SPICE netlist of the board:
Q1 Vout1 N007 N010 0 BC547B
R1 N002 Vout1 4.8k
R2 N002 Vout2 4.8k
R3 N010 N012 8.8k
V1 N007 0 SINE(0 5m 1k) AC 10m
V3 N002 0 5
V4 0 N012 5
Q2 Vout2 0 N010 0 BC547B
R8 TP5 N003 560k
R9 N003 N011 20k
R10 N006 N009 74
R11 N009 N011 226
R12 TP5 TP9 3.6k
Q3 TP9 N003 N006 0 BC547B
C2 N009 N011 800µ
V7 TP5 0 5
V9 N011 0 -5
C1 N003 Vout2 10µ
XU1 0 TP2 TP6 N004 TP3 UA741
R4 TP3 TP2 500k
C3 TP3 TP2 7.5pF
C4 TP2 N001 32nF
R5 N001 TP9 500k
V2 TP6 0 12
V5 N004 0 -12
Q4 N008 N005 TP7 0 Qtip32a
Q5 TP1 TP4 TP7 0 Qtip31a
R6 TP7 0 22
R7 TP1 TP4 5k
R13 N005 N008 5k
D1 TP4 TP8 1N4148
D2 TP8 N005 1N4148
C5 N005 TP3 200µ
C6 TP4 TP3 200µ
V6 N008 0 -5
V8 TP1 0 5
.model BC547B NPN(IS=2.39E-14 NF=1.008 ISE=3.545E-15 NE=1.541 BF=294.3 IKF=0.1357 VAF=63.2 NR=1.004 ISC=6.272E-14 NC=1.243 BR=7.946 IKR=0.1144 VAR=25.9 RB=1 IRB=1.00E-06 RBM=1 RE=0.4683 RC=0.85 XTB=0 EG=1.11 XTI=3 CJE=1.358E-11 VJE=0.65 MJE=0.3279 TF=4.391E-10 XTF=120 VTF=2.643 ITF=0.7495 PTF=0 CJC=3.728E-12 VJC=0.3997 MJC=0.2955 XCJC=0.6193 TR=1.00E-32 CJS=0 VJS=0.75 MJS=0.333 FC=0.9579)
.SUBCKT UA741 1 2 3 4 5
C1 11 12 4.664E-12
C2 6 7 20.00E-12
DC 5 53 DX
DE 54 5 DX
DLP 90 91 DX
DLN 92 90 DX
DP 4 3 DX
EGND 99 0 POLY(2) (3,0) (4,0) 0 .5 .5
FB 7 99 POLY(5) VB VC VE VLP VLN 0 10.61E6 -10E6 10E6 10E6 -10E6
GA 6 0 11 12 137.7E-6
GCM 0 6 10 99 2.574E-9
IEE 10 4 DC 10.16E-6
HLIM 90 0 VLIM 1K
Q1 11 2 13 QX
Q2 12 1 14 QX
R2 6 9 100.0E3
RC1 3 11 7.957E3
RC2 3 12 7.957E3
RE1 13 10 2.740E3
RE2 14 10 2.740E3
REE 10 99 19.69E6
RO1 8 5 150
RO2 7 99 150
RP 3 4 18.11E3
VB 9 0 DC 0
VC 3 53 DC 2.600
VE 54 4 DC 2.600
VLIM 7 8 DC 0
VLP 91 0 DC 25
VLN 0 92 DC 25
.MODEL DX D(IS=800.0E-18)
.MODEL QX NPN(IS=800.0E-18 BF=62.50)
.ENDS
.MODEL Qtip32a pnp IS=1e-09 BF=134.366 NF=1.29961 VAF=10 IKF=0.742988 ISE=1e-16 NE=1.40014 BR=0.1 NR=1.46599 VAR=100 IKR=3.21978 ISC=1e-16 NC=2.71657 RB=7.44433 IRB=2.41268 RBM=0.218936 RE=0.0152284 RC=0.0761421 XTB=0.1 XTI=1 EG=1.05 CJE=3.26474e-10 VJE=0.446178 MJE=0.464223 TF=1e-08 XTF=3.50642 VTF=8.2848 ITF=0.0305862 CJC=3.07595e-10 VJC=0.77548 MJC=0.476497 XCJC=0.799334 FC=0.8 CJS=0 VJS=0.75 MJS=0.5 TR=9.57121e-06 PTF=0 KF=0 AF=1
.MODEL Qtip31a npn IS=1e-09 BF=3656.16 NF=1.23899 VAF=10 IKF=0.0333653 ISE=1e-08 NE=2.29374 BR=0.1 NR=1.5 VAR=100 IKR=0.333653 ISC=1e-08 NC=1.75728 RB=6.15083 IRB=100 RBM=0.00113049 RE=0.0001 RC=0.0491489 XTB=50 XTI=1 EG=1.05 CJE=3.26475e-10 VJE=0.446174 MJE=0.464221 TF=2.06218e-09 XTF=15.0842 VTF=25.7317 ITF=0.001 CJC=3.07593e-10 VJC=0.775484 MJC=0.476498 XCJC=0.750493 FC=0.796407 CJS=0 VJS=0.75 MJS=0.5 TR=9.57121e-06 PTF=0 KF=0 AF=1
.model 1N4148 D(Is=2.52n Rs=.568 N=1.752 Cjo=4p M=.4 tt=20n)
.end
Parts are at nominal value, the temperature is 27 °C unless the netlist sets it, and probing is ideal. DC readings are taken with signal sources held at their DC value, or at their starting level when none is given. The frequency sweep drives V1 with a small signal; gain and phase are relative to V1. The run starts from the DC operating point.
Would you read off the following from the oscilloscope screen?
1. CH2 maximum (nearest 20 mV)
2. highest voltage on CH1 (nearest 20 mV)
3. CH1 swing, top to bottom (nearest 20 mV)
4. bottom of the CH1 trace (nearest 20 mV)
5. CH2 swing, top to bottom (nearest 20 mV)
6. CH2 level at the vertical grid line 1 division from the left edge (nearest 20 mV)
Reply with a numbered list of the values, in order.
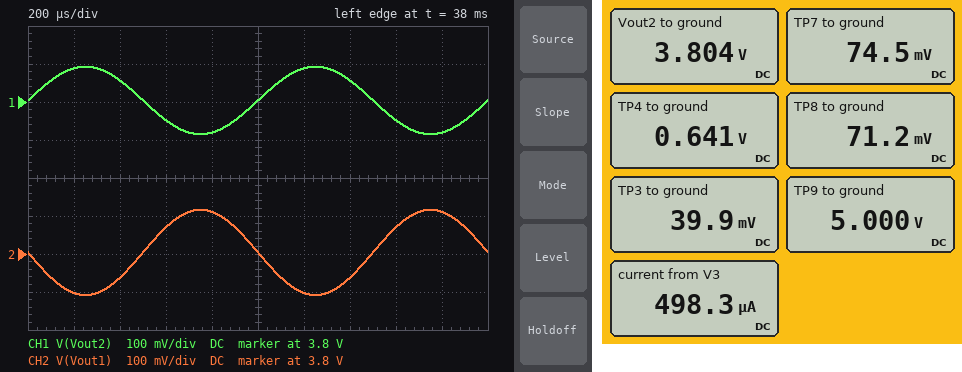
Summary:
1. 3.92 V
2. 3.90 V
3. 180 mV
4. 3.72 V
5. 220 mV
6. 3.70 V
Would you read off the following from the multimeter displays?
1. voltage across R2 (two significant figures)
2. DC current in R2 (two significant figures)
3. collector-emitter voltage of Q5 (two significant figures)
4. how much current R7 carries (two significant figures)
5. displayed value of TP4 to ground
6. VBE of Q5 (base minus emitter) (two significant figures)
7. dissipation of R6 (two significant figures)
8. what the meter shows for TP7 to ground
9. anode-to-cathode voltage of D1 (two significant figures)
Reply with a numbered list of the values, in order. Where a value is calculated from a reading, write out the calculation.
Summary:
1. 5 V - 3.804 V = 1.2 V
2. (5 V - 3.804 V) / 4.8 kΩ = 250 µA
3. 5 V - 74.5 mV = 4.9 V
4. (5 V - 641 mV) / 5 kΩ = 870 µA
5. 0.641 V
6. 641 mV - 74.5 mV = 570 mV
7. (74.5 mV)^2 / 22 Ω = 250 µW
8. 74.5 mV
9. 641 mV - 71.2 mV = 570 mV
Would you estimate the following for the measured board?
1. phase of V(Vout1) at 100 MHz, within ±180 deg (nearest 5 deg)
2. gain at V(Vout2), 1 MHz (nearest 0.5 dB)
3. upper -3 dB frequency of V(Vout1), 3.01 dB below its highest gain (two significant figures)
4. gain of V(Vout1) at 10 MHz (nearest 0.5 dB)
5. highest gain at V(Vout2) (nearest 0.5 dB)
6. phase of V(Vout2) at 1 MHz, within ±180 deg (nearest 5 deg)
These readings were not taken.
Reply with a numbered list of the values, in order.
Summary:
1. 85 deg
2. 24.0 dB
3. 18 MHz
4. 26.0 dB
5. 25.0 dB
6. -25 deg
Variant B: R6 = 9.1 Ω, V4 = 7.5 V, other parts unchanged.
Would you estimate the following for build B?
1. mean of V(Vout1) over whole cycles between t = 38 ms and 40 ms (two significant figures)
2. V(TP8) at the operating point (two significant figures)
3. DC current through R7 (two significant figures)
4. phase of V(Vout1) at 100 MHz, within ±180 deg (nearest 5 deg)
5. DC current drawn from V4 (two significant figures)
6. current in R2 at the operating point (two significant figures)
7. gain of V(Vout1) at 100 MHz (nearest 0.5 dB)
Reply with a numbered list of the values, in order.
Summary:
1. 3.1 V
2. 48 mV
3. 880 µA
4. 90 deg
5. 780 µA
6. 390 µA
7. 15.5 dB
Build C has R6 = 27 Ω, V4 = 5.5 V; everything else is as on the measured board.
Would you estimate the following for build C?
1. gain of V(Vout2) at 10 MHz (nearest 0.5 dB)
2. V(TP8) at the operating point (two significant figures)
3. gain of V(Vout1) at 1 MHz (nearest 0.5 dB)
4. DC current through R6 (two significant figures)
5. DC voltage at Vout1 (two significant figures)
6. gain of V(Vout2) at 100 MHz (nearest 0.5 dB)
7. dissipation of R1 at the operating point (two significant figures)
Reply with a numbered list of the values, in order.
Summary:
1. 12.0 dB
2. 76 mV
3. 28.0 dB
4. 2.9 mA
5. 3.7 V
6. -5.5 dB
7. 370 µW
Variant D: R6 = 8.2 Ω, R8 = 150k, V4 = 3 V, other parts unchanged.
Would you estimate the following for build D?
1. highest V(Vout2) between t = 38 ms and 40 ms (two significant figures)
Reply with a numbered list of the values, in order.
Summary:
1. 4.4 V
